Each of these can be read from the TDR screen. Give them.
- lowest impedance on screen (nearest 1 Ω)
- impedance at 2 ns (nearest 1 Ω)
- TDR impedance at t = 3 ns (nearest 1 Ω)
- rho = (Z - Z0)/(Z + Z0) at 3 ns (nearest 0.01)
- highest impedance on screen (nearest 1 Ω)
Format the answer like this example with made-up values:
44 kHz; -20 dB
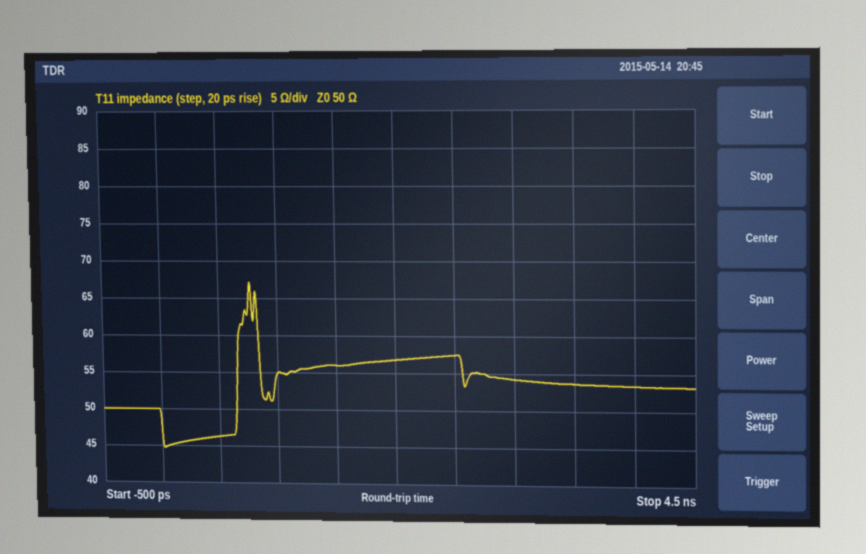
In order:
45 Ω; 57 Ω; 54 Ω; +0.04; 67 Ω
